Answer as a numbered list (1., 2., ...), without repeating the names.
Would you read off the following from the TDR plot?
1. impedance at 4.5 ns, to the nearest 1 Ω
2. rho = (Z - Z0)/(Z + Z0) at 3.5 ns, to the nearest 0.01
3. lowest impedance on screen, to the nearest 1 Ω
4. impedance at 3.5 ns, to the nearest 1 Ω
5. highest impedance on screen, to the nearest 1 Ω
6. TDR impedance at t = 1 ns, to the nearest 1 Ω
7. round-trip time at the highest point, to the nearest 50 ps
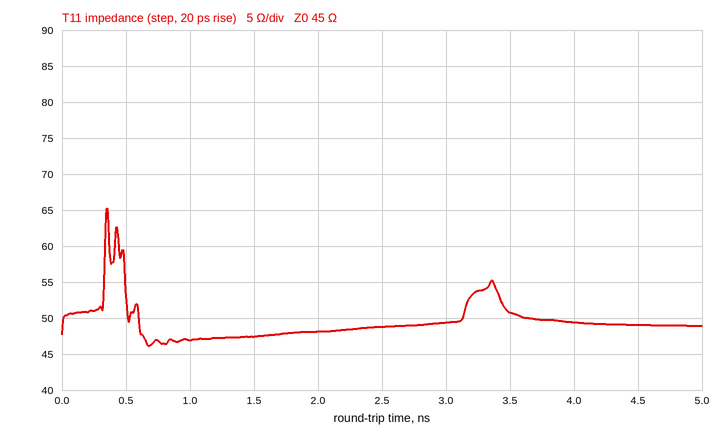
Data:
1. 49 Ω
2. +0.06
3. 46 Ω
4. 51 Ω
5. 65 Ω
6. 47 Ω
7. 350 ps
